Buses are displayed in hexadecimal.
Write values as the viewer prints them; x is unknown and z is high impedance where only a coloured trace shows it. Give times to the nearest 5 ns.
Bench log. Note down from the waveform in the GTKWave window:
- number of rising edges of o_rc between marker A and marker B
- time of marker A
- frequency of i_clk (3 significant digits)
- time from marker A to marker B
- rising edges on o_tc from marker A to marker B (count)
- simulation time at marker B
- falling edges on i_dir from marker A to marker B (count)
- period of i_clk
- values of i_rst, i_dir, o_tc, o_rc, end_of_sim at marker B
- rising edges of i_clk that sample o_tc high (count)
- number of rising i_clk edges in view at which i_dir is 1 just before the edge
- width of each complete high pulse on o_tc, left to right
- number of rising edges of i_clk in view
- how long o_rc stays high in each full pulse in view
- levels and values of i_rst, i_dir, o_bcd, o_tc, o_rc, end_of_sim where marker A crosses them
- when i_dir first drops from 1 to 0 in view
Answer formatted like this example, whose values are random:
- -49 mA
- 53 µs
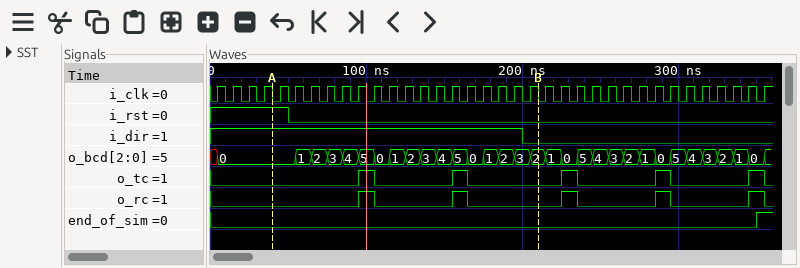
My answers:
- 2
- 40 ns
- 100 MHz
- 170 ns
- 2
- 210 ns
- 1
- 10 ns
- i_rst=0, i_dir=0, o_tc=0, o_rc=0, end_of_sim=0
- 5
- 20
- 10 ns, 10 ns, 10 ns, 10 ns, 10 ns
- 36
- 10 ns, 10 ns, 10 ns, 10 ns, 10 ns
- i_rst=1, i_dir=1, o_bcd=0, o_tc=0, o_rc=0, end_of_sim=0
- 200 ns
